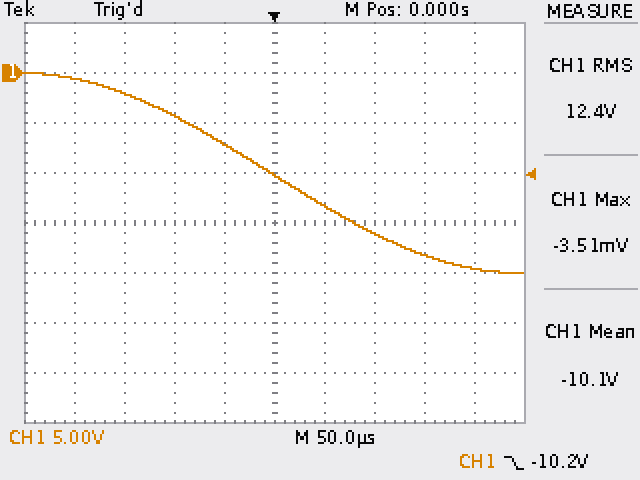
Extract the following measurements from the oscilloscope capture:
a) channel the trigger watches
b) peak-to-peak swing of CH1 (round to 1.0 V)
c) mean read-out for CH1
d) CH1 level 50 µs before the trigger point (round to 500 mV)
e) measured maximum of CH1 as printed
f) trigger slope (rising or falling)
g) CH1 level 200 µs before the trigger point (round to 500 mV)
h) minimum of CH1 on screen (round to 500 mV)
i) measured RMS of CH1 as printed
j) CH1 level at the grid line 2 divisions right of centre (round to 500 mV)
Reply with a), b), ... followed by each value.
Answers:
a) CH1
b) 20.0 V
c) -10.1 V
d) -7.0 V
e) -3.51 mV
f) falling
g) -500 mV
h) -20.0 V
i) 12.4 V
j) -16.0 V
